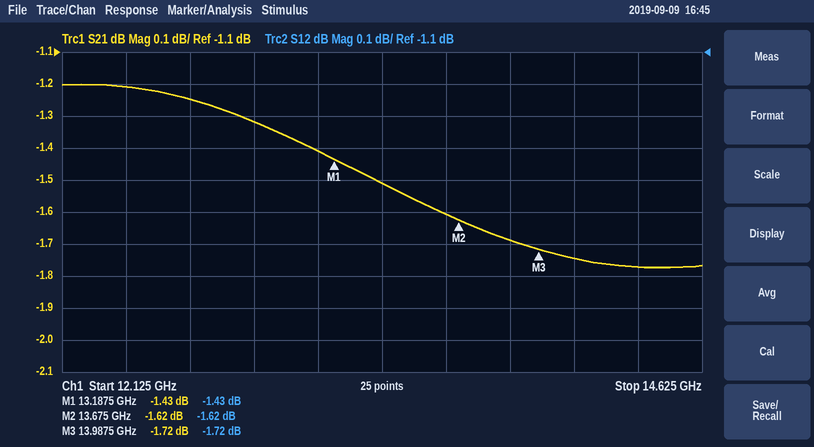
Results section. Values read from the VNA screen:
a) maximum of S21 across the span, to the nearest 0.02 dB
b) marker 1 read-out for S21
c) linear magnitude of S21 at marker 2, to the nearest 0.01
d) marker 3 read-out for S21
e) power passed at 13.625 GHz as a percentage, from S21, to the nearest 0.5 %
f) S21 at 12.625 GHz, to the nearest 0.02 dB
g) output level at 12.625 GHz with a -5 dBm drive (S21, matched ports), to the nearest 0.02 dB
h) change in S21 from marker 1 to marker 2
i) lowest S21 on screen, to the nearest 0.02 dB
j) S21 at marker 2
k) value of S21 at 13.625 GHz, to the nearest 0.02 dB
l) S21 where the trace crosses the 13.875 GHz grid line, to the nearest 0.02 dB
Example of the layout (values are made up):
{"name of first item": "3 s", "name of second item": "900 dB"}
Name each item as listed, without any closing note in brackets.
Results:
{"maximum of S21 across the span, to the nearest 0.02 dB": "-1.20 dB", "marker 1 read-out for S21": "-1.43 dB", "linear magnitude of S21 at marker 2, to the nearest 0.01": "0.83", "marker 3 read-out for S21": "-1.72 dB", "power passed at 13.625 GHz as a percentage, from S21, to the nearest 0.5 %": "69.0 %", "S21 at 12.625 GHz, to the nearest 0.02 dB": "-1.24 dB", "output level at 12.625 GHz with a -5 dBm drive (S21, matched ports), to the nearest 0.02 dB": "-6.24 dBm", "change in S21 from marker 1 to marker 2": "-0.19 dB", "lowest S21 on screen, to the nearest 0.02 dB": "-1.78 dB", "S21 at marker 2": "-1.62 dB", "value of S21 at 13.625 GHz, to the nearest 0.02 dB": "-1.60 dB", "S21 where the trace crosses the 13.875 GHz grid line, to the nearest 0.02 dB": "-1.68 dB"}
